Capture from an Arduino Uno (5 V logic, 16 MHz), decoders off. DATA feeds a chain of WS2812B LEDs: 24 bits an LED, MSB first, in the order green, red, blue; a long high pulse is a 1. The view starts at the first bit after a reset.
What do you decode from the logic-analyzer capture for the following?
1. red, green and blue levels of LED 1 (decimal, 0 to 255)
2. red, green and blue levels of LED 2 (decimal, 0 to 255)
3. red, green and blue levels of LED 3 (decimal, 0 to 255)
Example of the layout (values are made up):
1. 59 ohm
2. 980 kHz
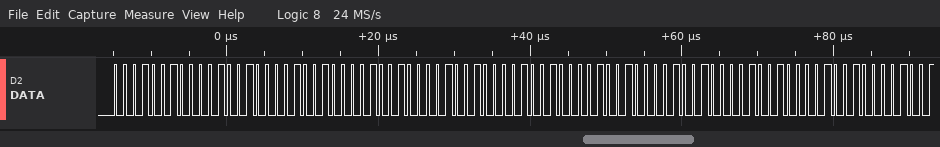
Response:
1. 18, 18, 18
2. 18, 18, 18
3. 18, 18, 18
